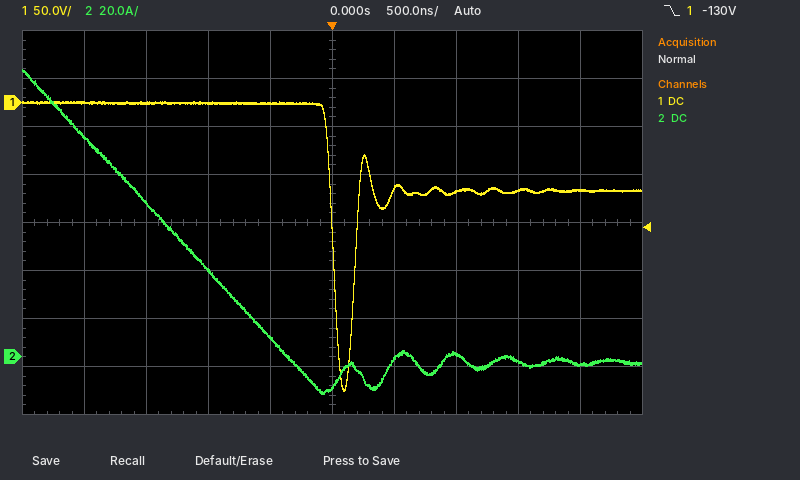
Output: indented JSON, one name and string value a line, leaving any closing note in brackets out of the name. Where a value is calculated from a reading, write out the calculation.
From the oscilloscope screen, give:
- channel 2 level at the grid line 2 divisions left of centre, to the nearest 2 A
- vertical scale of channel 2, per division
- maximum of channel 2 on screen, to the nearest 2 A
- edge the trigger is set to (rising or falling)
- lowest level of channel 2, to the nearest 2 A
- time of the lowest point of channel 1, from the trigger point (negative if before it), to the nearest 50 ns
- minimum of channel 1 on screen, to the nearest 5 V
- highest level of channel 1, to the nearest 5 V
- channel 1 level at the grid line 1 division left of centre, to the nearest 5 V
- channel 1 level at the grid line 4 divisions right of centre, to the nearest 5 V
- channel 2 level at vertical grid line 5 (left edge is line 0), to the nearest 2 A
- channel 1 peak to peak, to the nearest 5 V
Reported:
{
  "channel 2 level at the grid line 2 divisions left of centre, to the nearest 2 A": "36 A",
  "vertical scale of channel 2, per division": "20 A",
  "maximum of channel 2 on screen, to the nearest 2 A": "120 A",
  "edge the trigger is set to": "falling",
  "lowest level of channel 2, to the nearest 2 A": "-16 A",
  "time of the lowest point of channel 1, from the trigger point (negative if before it), to the nearest 50 ns": "+100 ns",
  "minimum of channel 1 on screen, to the nearest 5 V": "-300 V",
  "highest level of channel 1, to the nearest 5 V": "0 V",
  "channel 1 level at the grid line 1 division left of centre, to the nearest 5 V": "0 V",
  "channel 1 level at the grid line 4 divisions right of centre, to the nearest 5 V": "-90 V",
  "channel 2 level at vertical grid line 5 (left edge is line 0), to the nearest 2 A": "-12 A",
  "channel 1 peak to peak, to the nearest 5 V": "0 V − (-300 V) = 300 V"
}
